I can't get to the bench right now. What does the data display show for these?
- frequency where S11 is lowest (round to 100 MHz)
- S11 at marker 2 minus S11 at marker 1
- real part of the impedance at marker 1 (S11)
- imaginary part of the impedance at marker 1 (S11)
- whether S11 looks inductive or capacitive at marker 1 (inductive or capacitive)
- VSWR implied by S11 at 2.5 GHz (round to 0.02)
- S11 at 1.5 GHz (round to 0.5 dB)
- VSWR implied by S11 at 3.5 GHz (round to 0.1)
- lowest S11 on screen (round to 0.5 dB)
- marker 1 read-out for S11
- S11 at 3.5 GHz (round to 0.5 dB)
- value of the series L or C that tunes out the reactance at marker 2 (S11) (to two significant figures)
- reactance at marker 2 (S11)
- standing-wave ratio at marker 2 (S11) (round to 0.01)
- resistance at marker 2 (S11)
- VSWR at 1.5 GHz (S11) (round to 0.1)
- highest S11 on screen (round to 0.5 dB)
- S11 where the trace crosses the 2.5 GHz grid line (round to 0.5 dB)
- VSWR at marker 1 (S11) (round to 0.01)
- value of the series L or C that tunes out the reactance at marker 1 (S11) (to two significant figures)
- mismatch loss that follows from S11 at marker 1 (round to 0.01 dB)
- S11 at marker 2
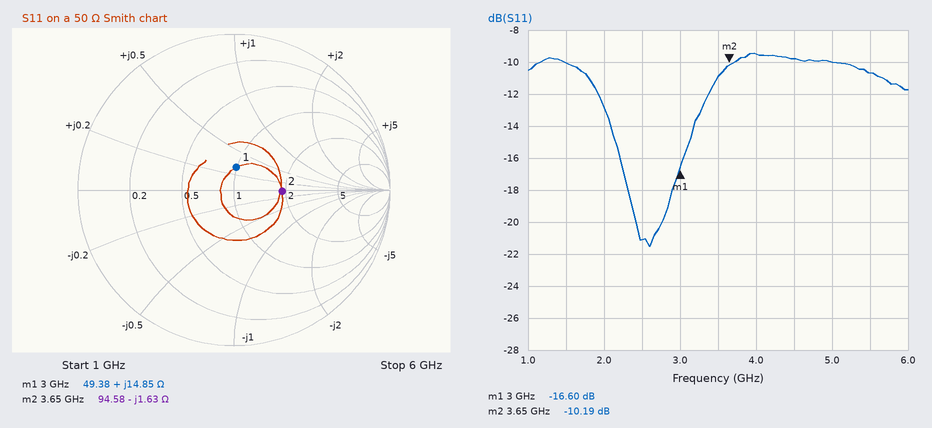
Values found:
2.6 GHz
6.41 dB
49.38 Ω
+14.85 Ω
inductive
1.20
-10.0 dB
1.8
-21.5 dB
-16.60 dB
-11.0 dB
71 pH
-1.63 Ω
1.89
94.58 Ω
1.9
-9.5 dB
-21.0 dB
1.35
3.6 pF
0.10 dB
-10.19 dB
